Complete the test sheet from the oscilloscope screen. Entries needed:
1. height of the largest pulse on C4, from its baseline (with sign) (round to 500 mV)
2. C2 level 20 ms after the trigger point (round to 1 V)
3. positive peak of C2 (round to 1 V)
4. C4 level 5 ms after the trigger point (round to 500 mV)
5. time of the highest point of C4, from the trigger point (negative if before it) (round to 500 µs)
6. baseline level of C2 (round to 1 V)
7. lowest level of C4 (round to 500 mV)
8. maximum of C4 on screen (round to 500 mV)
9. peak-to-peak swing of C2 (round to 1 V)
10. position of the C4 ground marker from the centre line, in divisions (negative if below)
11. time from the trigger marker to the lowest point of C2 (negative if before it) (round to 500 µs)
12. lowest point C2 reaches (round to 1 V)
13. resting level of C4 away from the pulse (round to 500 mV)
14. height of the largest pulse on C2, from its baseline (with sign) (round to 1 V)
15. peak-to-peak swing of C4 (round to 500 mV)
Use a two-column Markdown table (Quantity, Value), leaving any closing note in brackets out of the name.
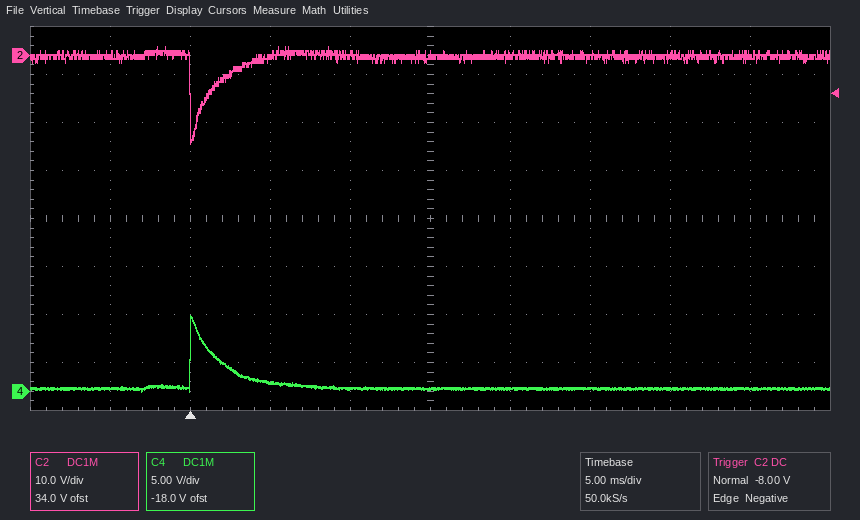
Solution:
| Quantity | Value |
|---|---|
| height of the largest pulse on C4, from its baseline (with sign) | +7.5 V |
| C2 level 20 ms after the trigger point | 0 V |
| positive peak of C2 | 2 V |
| C4 level 5 ms after the trigger point | 1.0 V |
| time of the highest point of C4, from the trigger point (negative if before it) | 0.0 ms |
| baseline level of C2 | 0 V |
| lowest level of C4 | 0.0 V |
| maximum of C4 on screen | 8.0 V |
| peak-to-peak swing of C2 | 20 V |
| position of the C4 ground marker from the centre line, in divisions | -3.6 div |
| time from the trigger marker to the lowest point of C2 (negative if before it) | 0.0 ms |
| lowest point C2 reaches | -18 V |
| resting level of C4 away from the pulse | 500 mV |
| height of the largest pulse on C2, from its baseline (with sign) | -18 V |
| peak-to-peak swing of C4 | 8.0 V |
